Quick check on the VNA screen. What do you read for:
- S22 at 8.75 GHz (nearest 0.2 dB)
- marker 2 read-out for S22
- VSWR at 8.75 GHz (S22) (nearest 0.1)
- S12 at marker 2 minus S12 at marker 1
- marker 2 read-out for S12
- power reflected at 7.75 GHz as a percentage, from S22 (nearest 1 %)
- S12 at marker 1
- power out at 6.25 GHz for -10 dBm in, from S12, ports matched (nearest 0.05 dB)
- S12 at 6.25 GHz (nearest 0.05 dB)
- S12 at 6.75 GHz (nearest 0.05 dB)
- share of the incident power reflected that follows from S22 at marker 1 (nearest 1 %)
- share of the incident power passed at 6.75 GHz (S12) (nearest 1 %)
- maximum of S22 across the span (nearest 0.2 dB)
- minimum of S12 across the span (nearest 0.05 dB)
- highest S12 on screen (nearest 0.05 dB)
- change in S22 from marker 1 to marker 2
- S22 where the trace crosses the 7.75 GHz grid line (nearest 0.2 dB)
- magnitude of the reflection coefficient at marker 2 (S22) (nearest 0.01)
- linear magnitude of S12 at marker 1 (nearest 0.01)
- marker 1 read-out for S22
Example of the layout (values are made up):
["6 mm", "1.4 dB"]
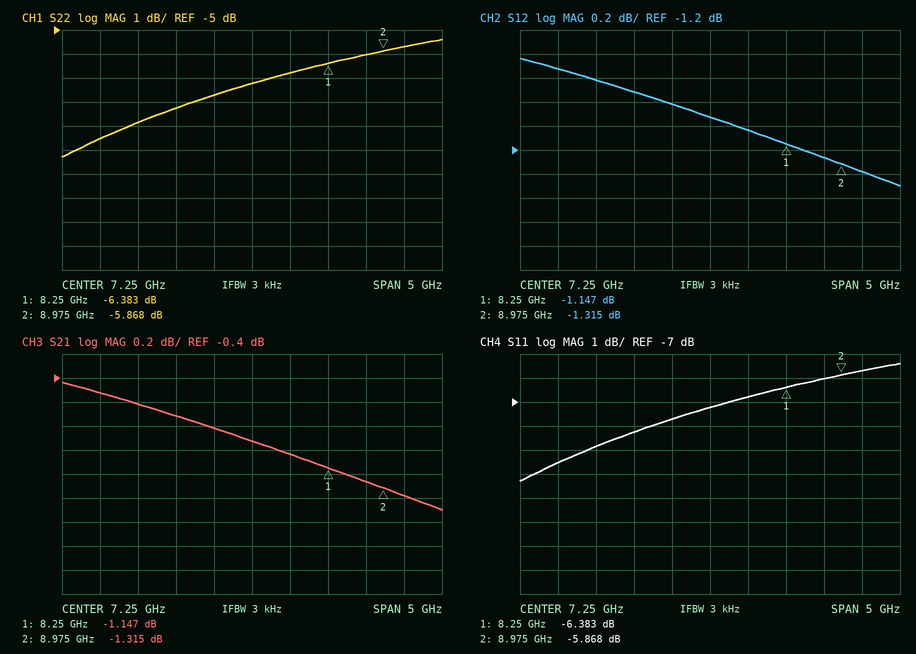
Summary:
["-6.0 dB", "-5.868 dB", "3.0", "-0.168 dB", "-1.315 dB", "21 %", "-1.147 dB", "-10.70 dBm", "-0.70 dB", "-0.80 dB", "23 %", "83 %", "-5.4 dB", "-1.50 dB", "-0.45 dB", "0.515 dB", "-6.8 dB", "0.51", "0.88", "-6.383 dB"]
